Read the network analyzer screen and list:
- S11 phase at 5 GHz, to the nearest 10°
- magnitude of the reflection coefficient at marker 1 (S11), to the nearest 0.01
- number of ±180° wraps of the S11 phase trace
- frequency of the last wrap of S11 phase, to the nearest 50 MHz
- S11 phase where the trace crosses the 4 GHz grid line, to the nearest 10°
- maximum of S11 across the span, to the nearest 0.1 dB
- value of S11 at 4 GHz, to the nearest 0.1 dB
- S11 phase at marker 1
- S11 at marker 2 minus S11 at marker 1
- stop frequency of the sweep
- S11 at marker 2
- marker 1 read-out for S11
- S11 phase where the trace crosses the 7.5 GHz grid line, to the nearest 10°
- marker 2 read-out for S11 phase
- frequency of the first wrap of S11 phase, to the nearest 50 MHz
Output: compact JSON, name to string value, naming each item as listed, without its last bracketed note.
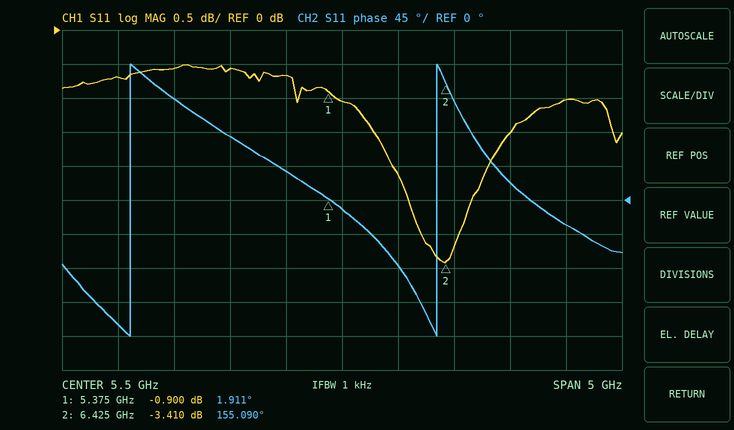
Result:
{"S11 phase at 5 GHz, to the nearest 10°": "40°", "magnitude of the reflection coefficient at marker 1 (S11), to the nearest 0.01": "0.90", "number of ±180° wraps of the S11 phase trace": "2", "frequency of the last wrap of S11 phase, to the nearest 50 MHz": "6.35 GHz", "S11 phase where the trace crosses the 4 GHz grid line, to the nearest 10°": "130°", "maximum of S11 across the span, to the nearest 0.1 dB": "-0.5 dB", "value of S11 at 4 GHz, to the nearest 0.1 dB": "-0.6 dB", "S11 phase at marker 1": "1.911°", "S11 at marker 2 minus S11 at marker 1": "-2.510 dB", "stop frequency of the sweep": "8 GHz", "S11 at marker 2": "-3.410 dB", "marker 1 read-out for S11": "-0.900 dB", "S11 phase where the trace crosses the 7.5 GHz grid line, to the nearest 10°": "-30°", "marker 2 read-out for S11 phase": "155.090°", "frequency of the first wrap of S11 phase, to the nearest 50 MHz": "3.60 GHz"}
